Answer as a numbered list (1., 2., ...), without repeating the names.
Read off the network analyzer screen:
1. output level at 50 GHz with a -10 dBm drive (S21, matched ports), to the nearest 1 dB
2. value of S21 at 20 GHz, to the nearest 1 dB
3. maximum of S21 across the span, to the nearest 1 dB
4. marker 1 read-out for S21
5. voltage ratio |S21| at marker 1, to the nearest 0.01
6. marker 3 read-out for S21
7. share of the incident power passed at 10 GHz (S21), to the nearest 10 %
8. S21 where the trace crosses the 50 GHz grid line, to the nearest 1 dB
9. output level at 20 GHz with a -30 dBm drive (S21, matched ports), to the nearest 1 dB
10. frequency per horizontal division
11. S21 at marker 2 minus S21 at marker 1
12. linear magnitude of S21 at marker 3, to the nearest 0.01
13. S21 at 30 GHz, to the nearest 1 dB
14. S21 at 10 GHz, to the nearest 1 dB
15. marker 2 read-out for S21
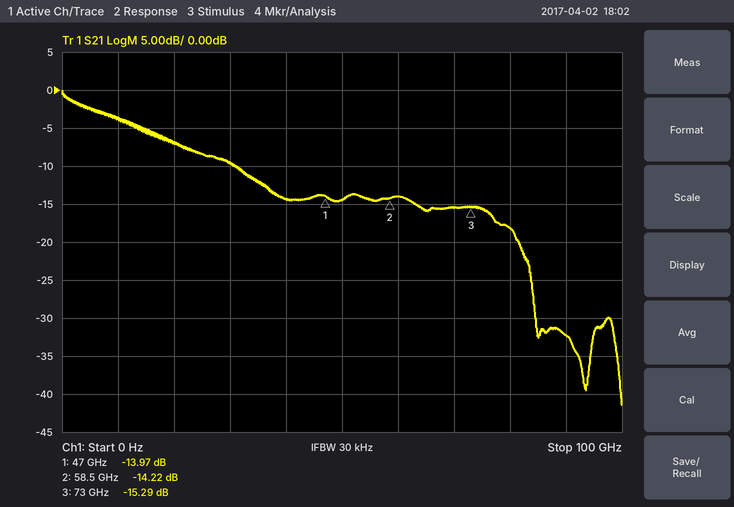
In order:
1. -24 dBm
2. -7 dB
3. 0 dB
4. -13.97 dB
5. 0.20
6. -15.29 dB
7. 40 %
8. -14 dB
9. -37 dBm
10. 10 GHz
11. -0.25 dB
12. 0.17
13. -10 dB
14. -4 dB
15. -14.22 dB
